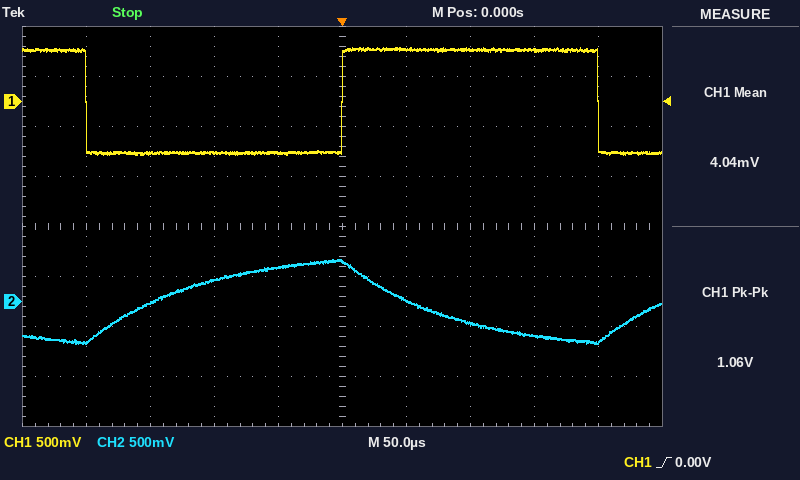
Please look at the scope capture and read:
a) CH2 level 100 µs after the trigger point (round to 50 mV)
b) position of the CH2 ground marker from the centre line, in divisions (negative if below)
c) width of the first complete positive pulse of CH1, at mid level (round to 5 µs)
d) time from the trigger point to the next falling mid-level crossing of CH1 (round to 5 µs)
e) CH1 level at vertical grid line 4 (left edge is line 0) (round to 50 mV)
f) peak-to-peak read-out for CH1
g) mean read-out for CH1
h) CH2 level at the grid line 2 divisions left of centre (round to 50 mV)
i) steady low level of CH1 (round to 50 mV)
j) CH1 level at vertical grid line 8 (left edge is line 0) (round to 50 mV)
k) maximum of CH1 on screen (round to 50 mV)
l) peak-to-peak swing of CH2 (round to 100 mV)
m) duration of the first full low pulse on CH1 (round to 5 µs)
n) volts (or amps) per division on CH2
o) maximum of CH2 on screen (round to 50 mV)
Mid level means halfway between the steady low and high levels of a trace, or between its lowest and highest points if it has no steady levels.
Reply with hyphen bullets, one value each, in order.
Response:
- -200 mV
- -1.5 div
- 200 µs
- 200 µs
- -500 mV
- 1.06 V
- 4.04 mV
- 200 mV
- -500 mV
- 500 mV
- 550 mV
- 800 mV
- 200 µs
- 500 mV
- 400 mV
